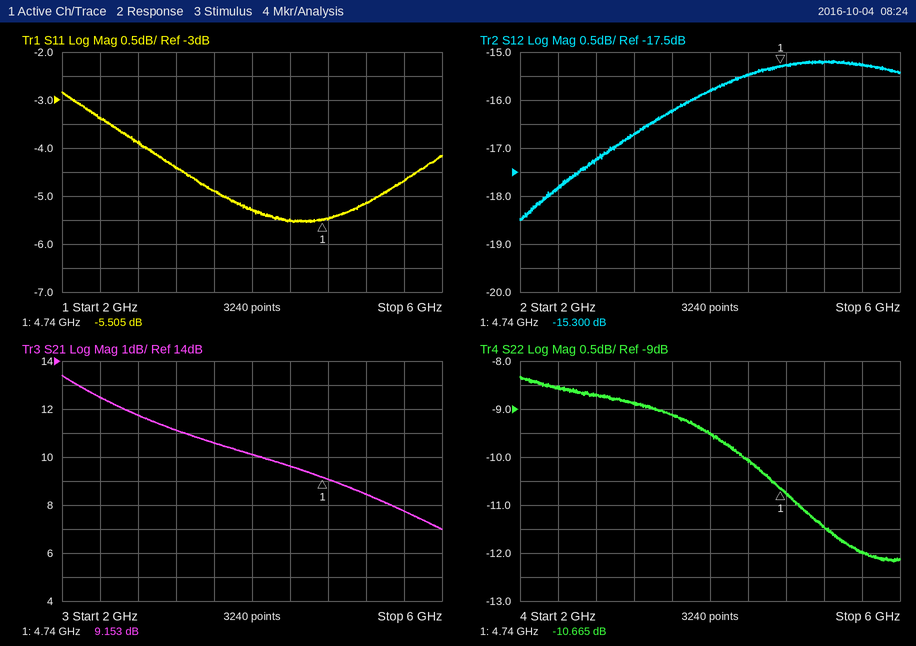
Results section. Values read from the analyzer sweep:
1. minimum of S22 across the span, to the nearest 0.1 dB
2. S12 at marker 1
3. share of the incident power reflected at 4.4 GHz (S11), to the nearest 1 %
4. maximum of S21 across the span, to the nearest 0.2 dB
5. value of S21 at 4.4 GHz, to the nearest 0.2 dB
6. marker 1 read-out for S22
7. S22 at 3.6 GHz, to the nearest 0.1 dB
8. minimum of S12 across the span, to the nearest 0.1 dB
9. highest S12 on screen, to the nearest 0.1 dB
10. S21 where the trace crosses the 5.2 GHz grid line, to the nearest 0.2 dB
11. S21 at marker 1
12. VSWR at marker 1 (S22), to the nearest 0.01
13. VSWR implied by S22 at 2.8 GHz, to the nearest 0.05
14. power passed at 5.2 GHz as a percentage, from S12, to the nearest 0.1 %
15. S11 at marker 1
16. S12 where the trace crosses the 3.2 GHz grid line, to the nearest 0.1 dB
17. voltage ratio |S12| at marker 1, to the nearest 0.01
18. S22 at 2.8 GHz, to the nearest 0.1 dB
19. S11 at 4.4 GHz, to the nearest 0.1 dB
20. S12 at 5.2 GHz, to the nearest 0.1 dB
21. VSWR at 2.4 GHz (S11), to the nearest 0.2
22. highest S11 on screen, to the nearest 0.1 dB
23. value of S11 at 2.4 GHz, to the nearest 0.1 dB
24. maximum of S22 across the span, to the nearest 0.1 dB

-12.2 dB
-15.300 dB
28 %
13.4 dB
9.6 dB
-10.665 dB
-9.1 dB
-18.5 dB
-15.2 dB
8.4 dB
9.153 dB
1.83
2.15
3.0 %
-5.505 dB
-16.7 dB
0.17
-8.7 dB
-5.5 dB
-15.2 dB
5.2
-2.8 dB
-3.4 dB
-8.3 dB
